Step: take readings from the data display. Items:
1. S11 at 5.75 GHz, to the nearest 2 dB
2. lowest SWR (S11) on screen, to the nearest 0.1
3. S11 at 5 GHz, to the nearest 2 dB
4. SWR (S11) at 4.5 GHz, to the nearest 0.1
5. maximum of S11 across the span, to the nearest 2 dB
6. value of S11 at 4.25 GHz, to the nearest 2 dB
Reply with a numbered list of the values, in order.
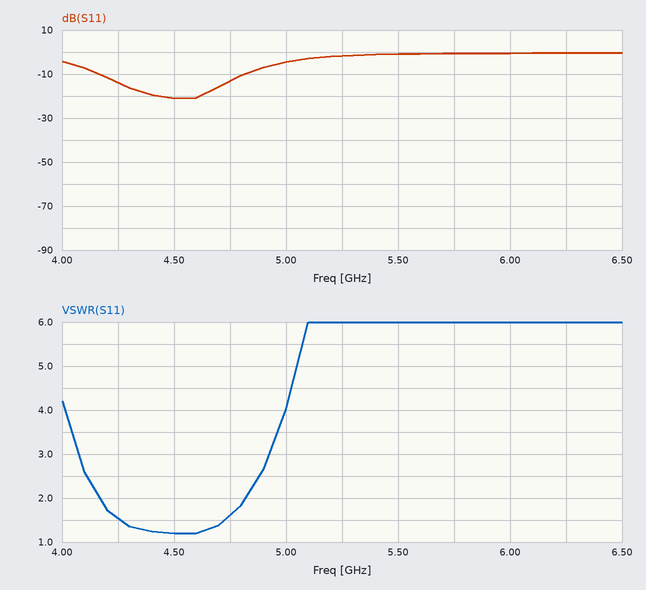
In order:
1. 0 dB
2. 1.2
3. -4 dB
4. 1.2
5. 0 dB
6. -14 dB
